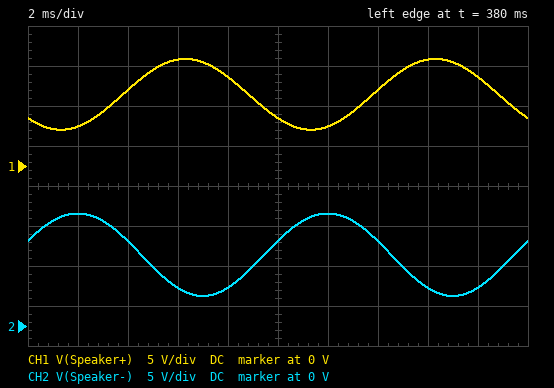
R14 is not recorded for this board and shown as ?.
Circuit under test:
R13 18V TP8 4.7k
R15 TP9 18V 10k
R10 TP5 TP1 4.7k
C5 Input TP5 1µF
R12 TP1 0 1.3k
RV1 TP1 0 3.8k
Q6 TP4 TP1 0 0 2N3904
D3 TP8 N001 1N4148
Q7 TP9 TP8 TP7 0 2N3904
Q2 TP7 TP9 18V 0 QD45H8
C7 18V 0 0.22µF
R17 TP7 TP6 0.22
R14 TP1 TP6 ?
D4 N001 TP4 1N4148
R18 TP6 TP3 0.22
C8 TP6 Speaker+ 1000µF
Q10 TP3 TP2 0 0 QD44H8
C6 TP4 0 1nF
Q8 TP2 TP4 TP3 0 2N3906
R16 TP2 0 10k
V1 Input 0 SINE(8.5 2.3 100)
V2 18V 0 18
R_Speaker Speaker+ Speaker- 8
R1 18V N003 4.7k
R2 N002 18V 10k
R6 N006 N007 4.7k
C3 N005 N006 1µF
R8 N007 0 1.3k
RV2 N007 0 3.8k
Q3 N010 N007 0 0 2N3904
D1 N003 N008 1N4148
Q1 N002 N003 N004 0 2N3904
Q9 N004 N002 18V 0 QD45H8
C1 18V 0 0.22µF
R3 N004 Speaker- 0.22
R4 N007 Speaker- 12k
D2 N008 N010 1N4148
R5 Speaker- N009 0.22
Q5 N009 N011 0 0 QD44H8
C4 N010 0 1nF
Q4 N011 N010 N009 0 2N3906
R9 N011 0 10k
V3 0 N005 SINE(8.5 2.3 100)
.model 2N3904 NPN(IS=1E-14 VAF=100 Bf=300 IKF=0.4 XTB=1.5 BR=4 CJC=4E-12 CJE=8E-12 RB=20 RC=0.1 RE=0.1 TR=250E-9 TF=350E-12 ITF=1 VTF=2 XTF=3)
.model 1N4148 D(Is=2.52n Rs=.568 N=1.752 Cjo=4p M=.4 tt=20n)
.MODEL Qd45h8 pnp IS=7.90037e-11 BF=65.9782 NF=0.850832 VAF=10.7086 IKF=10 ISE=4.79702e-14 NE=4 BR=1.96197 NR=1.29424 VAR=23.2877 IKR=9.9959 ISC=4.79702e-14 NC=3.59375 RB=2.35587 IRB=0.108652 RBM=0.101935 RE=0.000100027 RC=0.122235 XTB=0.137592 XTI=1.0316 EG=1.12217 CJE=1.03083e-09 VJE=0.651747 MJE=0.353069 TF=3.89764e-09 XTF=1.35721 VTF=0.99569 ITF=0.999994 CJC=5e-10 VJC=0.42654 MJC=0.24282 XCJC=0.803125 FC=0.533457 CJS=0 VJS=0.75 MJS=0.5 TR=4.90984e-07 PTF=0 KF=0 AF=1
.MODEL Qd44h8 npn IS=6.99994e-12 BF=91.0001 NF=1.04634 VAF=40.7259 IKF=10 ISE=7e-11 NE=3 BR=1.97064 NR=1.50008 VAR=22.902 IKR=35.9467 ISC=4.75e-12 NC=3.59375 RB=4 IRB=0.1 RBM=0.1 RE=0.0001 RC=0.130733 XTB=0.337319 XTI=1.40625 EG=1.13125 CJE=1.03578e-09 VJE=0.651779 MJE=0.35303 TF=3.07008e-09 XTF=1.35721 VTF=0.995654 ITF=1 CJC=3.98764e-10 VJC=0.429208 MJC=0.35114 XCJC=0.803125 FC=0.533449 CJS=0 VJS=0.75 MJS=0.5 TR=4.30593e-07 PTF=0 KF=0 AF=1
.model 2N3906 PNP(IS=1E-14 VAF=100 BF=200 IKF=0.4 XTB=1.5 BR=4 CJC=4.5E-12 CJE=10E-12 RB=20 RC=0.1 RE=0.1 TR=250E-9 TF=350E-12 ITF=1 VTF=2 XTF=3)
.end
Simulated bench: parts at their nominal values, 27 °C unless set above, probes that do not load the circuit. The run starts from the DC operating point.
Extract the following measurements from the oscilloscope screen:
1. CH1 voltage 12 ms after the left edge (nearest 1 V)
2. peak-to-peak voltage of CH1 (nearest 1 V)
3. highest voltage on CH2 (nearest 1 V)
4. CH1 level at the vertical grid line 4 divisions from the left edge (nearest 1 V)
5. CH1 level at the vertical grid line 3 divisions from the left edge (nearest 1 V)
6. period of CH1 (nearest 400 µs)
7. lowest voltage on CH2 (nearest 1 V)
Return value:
5 V
9 V
14 V
11 V
13 V
10.0 ms
4 V
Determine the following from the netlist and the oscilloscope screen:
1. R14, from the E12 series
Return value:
10 kΩ
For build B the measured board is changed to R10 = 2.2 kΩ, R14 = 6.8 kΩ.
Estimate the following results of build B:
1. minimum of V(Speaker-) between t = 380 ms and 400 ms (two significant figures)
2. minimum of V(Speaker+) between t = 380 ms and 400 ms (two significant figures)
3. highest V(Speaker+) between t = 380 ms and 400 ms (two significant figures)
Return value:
3.8 V
3.3 V
15 V
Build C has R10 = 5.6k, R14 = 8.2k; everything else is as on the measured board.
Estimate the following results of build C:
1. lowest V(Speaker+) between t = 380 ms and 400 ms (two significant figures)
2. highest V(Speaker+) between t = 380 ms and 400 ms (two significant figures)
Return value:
5.8 V
12 V
